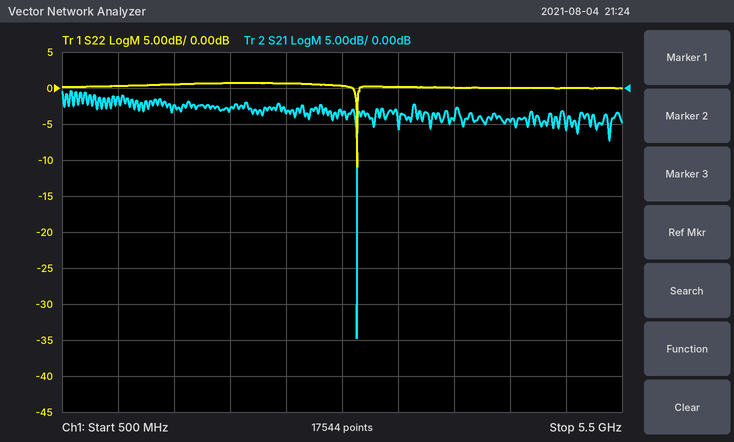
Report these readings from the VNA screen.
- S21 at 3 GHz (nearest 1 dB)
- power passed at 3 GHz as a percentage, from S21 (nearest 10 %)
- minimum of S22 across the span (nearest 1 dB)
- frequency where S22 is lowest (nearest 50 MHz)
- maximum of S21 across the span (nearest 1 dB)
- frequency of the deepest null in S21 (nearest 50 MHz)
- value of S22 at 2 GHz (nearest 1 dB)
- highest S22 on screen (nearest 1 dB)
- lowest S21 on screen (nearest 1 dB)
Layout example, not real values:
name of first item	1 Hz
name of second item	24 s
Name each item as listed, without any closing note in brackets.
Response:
S21 at 3 GHz	-4 dB
power passed at 3 GHz as a percentage, from S21	40 %
minimum of S22 across the span	-11 dB
frequency where S22 is lowest	3.15 GHz
maximum of S21 across the span	0 dB
frequency of the deepest null in S21	3.15 GHz
value of S22 at 2 GHz	1 dB
highest S22 on screen	1 dB
lowest S21 on screen	-35 dB
